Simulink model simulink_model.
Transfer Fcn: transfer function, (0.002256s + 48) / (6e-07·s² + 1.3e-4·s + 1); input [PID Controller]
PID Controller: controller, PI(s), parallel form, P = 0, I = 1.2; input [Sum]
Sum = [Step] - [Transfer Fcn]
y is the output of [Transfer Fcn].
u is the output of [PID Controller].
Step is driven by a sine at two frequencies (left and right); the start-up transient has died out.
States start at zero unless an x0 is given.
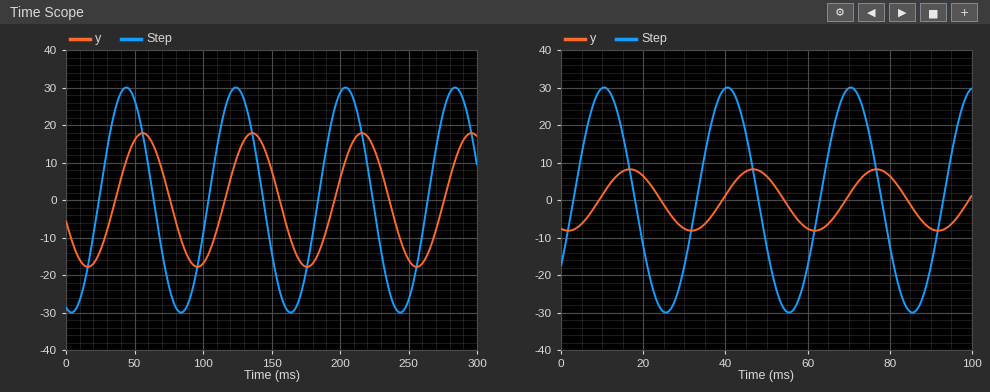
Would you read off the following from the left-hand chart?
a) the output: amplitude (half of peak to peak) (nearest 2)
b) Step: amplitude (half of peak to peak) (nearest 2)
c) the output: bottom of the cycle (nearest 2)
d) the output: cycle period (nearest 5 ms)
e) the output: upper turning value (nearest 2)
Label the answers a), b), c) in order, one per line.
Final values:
a) 18
b) 30
c) -18
d) 80 ms
e) 18
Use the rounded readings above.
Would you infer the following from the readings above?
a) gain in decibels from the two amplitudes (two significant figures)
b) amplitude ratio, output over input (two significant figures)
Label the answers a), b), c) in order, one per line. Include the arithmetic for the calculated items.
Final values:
a) 20 log10(18 / 30) = -4.4 dB
b) 18 / 30 = 0.60
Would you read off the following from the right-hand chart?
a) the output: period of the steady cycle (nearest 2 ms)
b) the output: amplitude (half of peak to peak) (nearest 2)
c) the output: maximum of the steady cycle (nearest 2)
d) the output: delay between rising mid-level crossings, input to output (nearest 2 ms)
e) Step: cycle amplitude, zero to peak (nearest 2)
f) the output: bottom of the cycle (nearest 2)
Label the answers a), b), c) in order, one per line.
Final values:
a) 30 ms
b) 8
c) 8
d) 6 ms
e) 30
f) -8
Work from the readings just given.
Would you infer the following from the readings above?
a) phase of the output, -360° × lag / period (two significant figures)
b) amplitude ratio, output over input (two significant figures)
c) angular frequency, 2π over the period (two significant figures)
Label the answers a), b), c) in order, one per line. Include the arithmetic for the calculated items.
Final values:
a) -360 × 6 / 30 = -72°
b) 8 / 30 = 0.27
c) 2π / 30 = 0.21 rad/ms
